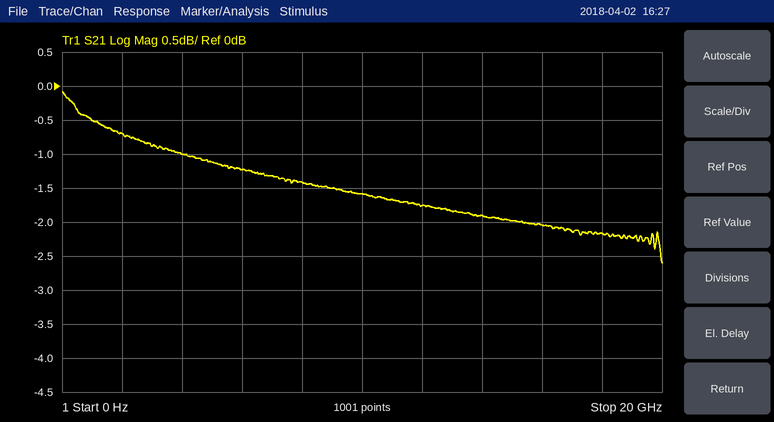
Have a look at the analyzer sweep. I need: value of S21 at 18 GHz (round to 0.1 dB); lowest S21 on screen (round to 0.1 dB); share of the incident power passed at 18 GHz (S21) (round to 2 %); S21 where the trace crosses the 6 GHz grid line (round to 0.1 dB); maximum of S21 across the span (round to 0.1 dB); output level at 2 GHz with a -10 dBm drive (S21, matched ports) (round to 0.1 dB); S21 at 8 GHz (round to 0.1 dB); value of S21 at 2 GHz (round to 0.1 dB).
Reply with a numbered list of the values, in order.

1. -2.2 dB
2. -2.6 dB
3. 60 %
4. -1.2 dB
5. -0.1 dB
6. -10.7 dBm
7. -1.4 dB
8. -0.7 dB
